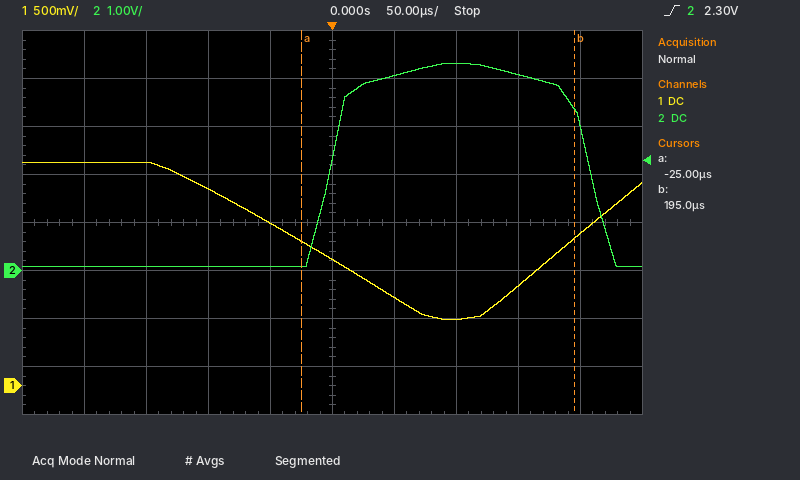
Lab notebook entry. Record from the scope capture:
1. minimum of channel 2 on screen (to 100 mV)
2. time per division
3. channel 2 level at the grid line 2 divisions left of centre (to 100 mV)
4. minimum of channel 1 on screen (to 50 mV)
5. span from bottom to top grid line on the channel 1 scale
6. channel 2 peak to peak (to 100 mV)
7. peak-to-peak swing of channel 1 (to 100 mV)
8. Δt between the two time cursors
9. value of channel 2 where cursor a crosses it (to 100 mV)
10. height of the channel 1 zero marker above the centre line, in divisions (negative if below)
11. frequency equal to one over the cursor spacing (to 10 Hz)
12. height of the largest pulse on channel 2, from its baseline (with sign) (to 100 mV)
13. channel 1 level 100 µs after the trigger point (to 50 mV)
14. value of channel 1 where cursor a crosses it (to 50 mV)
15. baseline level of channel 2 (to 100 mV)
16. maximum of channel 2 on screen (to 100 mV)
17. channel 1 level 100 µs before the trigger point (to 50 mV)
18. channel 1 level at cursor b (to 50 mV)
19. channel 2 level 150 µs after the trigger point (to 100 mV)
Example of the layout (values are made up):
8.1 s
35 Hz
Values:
100 mV
50 µs
100 mV
700 mV
4 V
4.2 V
1.60 V
220 µs
100 mV
-3.4 div
4.55 kHz
+4.2 V
700 mV
1.50 V
100 mV
4.3 V
2.05 V
1.55 V
4.1 V
